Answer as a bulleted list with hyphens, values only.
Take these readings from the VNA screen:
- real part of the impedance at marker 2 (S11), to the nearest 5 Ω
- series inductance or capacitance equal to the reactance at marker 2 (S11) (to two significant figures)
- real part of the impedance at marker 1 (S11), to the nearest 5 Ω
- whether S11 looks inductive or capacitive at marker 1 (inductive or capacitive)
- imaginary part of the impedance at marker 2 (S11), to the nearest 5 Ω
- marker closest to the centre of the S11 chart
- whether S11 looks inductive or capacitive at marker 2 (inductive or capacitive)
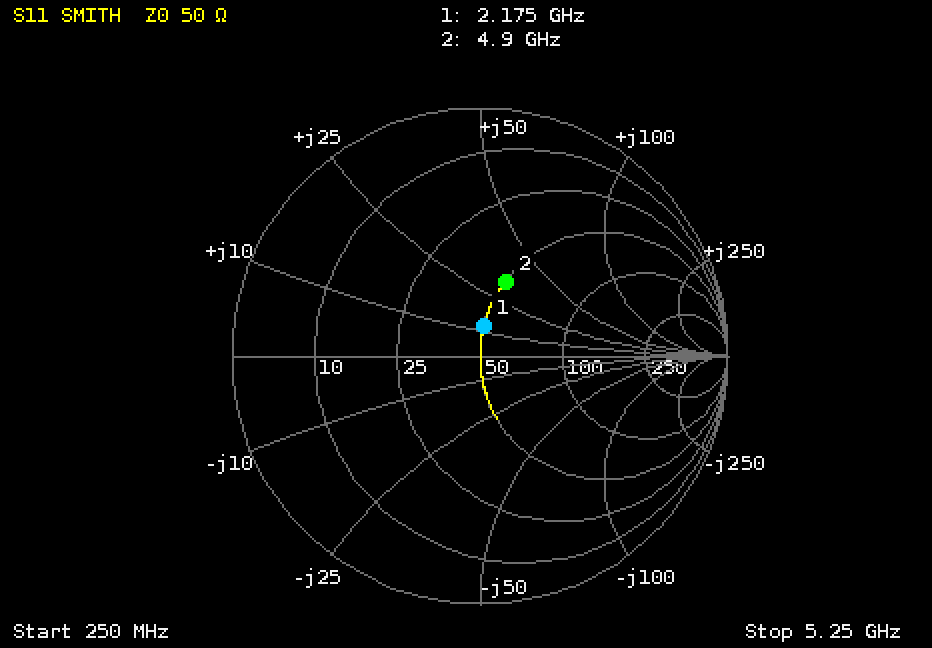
- 50 Ω
- 1.1 nH
- 50 Ω
- inductive
- +35 Ω
- marker 1
- inductive
